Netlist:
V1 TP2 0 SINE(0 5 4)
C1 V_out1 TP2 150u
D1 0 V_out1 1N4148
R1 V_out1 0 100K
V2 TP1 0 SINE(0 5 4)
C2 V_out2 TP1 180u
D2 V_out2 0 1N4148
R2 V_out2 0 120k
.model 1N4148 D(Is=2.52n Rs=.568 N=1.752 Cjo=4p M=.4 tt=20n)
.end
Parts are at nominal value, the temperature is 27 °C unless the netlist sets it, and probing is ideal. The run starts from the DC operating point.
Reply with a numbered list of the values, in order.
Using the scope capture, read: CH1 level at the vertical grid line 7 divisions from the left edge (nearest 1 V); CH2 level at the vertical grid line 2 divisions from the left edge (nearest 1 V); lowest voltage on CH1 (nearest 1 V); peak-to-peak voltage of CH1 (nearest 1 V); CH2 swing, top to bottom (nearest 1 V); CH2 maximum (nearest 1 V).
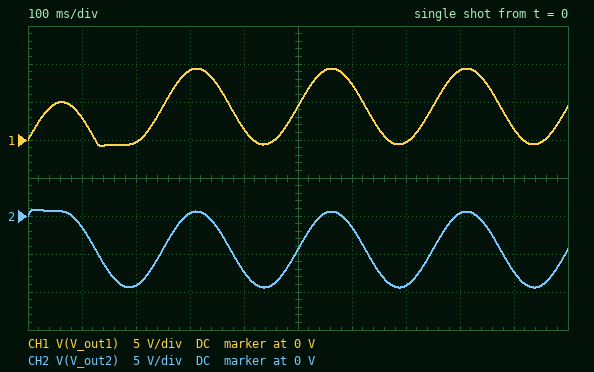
1. 0 V
2. -9 V
3. -1 V
4. 10 V
5. 10 V
6. 1 V
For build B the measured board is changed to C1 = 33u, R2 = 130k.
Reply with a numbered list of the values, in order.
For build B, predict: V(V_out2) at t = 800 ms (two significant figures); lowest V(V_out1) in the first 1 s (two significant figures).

1. 360 mV
2. -650 mV
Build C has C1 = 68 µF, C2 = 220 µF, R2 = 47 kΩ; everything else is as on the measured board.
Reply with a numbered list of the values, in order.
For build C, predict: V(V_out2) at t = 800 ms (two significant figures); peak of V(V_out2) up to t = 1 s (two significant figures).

1. 440 mV
2. 750 mV
